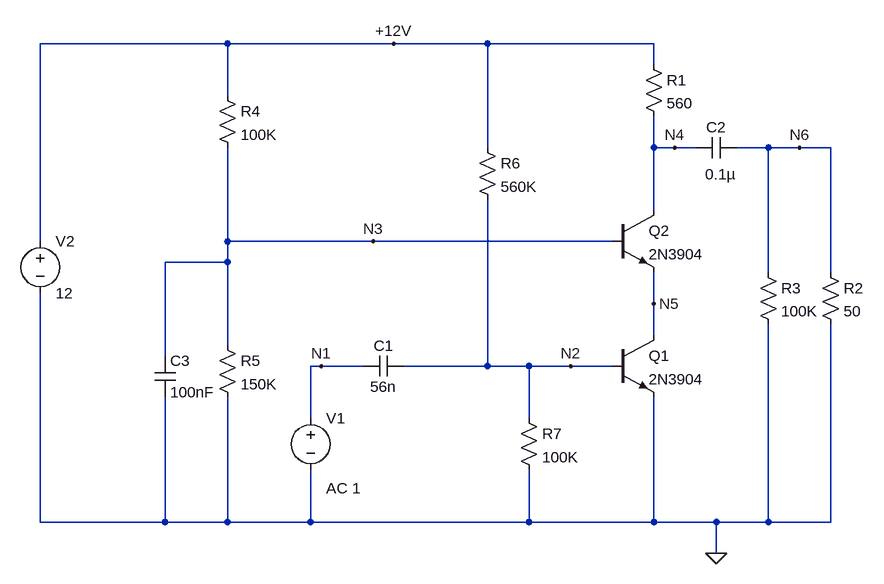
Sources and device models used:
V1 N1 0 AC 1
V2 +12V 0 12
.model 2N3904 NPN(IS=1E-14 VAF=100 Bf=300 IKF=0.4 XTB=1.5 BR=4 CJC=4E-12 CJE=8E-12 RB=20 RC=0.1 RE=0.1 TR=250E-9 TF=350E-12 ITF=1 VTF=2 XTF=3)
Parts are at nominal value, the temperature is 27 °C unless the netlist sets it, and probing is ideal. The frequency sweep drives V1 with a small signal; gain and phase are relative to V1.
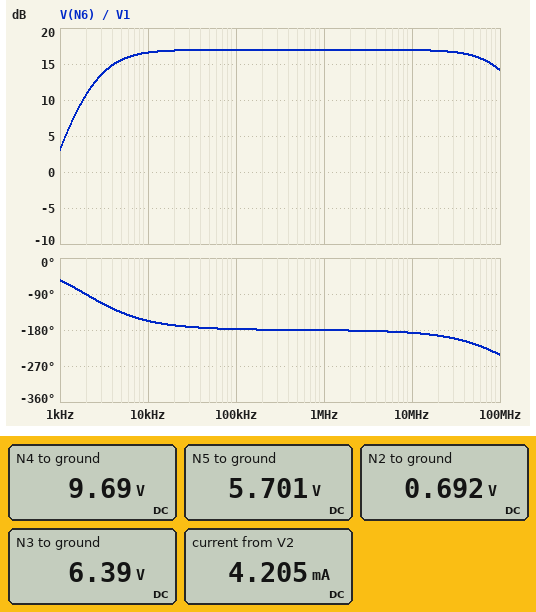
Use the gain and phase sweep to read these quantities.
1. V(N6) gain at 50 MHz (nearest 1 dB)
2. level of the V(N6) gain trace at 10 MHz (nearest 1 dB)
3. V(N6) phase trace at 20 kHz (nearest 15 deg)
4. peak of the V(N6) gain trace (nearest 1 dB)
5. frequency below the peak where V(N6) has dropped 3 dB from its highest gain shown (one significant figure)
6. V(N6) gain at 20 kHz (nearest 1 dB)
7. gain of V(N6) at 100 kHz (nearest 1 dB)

16 dB
17 dB
-165 deg
17 dB
3 kHz
17 dB
17 dB
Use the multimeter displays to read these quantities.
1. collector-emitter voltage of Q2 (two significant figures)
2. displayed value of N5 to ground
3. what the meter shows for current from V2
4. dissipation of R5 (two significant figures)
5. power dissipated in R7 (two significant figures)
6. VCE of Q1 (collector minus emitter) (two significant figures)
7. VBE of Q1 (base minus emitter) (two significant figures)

4.0 V
5.701 V
4.205 mA
270 µW
4.8 µW
5.7 V
690 mV
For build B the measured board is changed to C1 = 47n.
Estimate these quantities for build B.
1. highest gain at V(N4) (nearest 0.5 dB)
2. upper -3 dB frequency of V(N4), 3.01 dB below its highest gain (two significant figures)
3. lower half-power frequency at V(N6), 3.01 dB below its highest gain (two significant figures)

34.5 dB
5.3 kHz
3.4 kHz
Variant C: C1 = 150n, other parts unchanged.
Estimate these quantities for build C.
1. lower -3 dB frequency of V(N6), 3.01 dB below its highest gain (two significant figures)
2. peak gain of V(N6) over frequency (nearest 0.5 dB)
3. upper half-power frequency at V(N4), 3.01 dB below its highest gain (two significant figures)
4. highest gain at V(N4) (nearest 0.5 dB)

2.7 kHz
17.0 dB
3.6 kHz
37.0 dB
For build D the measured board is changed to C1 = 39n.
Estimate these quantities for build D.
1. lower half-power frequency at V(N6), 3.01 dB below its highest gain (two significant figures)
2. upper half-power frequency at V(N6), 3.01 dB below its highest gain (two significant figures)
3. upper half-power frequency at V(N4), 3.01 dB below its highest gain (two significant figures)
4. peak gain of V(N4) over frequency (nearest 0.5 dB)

3.7 kHz
100 MHz
5.8 kHz
33.5 dB
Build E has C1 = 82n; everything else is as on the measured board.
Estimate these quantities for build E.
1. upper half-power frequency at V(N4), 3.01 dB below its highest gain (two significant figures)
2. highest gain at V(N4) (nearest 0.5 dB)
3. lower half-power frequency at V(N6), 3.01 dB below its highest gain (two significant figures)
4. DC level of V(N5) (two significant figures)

4.3 kHz
36.0 dB
2.9 kHz
5.7 V
